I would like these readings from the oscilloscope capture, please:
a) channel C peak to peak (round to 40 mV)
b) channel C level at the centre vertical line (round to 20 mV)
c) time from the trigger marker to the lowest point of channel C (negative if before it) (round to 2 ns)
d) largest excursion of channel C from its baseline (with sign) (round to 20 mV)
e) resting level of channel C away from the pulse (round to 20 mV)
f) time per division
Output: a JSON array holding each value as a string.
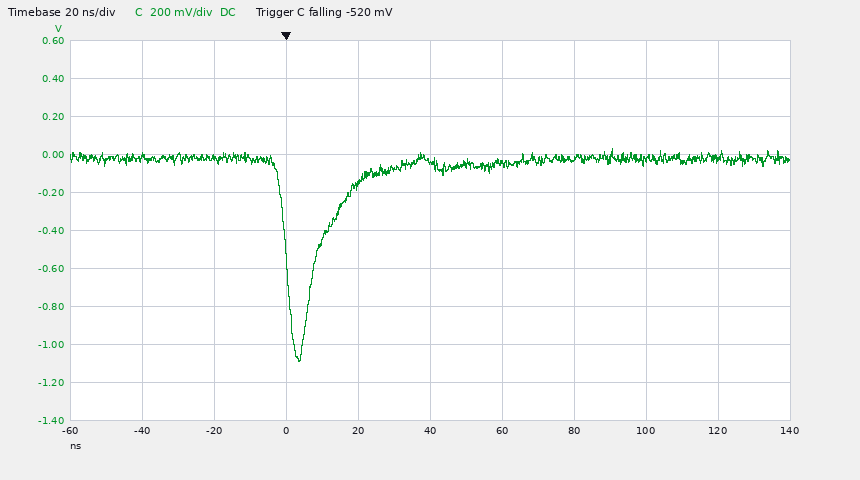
["1.12 V", "-40 mV", "+4 ns", "-1.06 V", "-20 mV", "20 ns"]
